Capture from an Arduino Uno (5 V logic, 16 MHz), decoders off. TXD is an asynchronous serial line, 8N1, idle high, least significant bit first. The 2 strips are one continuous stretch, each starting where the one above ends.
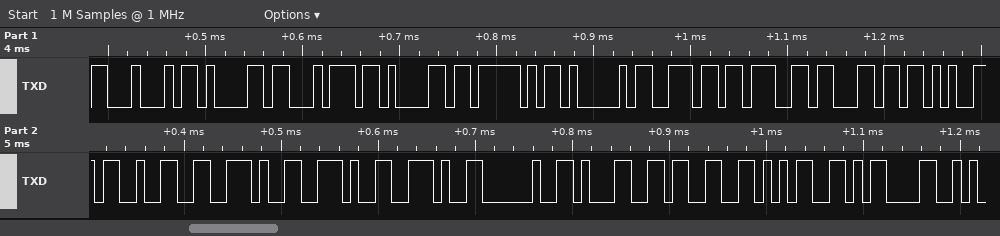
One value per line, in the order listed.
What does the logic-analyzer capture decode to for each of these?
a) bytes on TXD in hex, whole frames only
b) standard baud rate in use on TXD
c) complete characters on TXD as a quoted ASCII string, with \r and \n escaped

44 61 74 61 5F 41 6E 67 6C 65 32 2E 2E 2E 20 31 33 35 0D
115200 baud
"Data_Angle2... 135\r"
